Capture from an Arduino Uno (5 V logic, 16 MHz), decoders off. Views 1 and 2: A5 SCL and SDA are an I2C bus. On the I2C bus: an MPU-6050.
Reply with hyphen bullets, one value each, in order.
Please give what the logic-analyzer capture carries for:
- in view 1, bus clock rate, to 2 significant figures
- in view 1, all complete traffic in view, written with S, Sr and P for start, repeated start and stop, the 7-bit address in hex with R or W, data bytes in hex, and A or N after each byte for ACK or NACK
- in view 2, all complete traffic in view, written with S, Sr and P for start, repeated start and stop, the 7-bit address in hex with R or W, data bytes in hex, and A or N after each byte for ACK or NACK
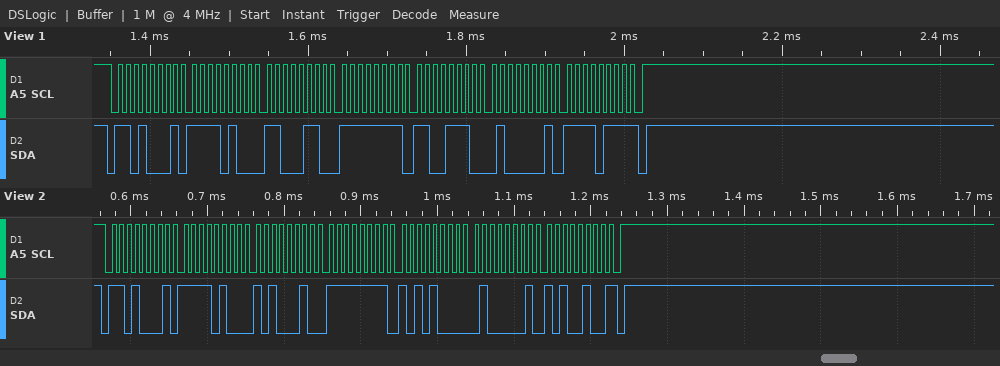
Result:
- 100 kHz
- S 68R A F4 A C6 A FF A CE A 41 A F7 N P
- S 68R A F4 A A2 A FF A A8 A 41 A A4 N P
